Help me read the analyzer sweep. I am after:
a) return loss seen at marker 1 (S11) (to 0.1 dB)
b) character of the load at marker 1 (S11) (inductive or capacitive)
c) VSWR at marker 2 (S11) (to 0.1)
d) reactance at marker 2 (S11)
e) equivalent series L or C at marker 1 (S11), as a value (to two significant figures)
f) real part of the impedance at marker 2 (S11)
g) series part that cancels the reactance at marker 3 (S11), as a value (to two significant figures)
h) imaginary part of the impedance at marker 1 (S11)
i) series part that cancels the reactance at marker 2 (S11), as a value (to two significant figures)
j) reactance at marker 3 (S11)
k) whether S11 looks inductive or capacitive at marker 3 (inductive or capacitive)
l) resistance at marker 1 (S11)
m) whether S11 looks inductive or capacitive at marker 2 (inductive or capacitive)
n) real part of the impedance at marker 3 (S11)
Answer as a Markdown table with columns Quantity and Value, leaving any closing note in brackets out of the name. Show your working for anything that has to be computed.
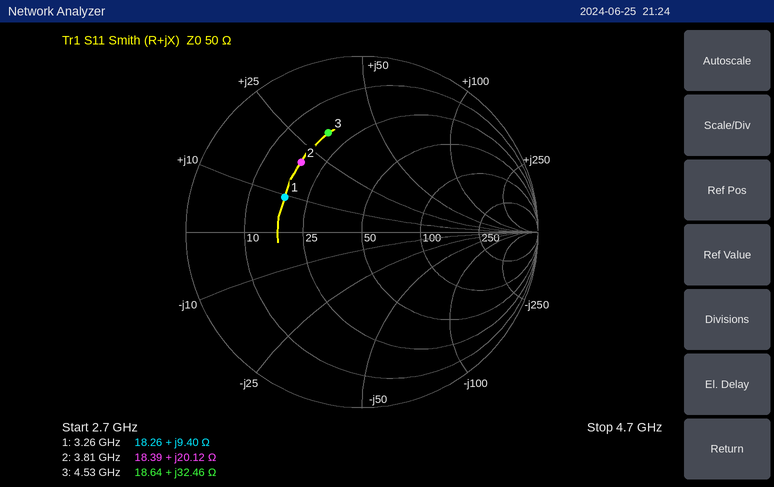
| Quantity | Value |
|---|---|
| return loss seen at marker 1 (S11) | 6.4 dB |
| character of the load at marker 1 (S11) | inductive |
| VSWR at marker 2 (S11) | 3.2 |
| reactance at marker 2 | +20.12 Ω |
| equivalent series L or C at marker 1 (S11), as a value | L = 9.4 Ω/(2π × 3.26 GHz) ≈ 459 pH, so 460 pH to two significant figures |
| real part of the impedance at marker 2 | 18.39 Ω |
| series part that cancels the reactance at marker 3 (S11), as a value | C = 1/(2π × 4.53 GHz × 32.46 Ω) ≈ 1.1 pF |
| imaginary part of the impedance at marker 1 | +9.40 Ω |
| series part that cancels the reactance at marker 2 (S11), as a value | C = 1/(2π × 3.81 GHz × 20.12 Ω) ≈ 2.1 pF |
| reactance at marker 3 | +32.46 Ω |
| whether S11 looks inductive or capacitive at marker 3 | inductive |
| resistance at marker 1 | 18.26 Ω |
| whether S11 looks inductive or capacitive at marker 2 | inductive |
| real part of the impedance at marker 3 | 18.64 Ω |
